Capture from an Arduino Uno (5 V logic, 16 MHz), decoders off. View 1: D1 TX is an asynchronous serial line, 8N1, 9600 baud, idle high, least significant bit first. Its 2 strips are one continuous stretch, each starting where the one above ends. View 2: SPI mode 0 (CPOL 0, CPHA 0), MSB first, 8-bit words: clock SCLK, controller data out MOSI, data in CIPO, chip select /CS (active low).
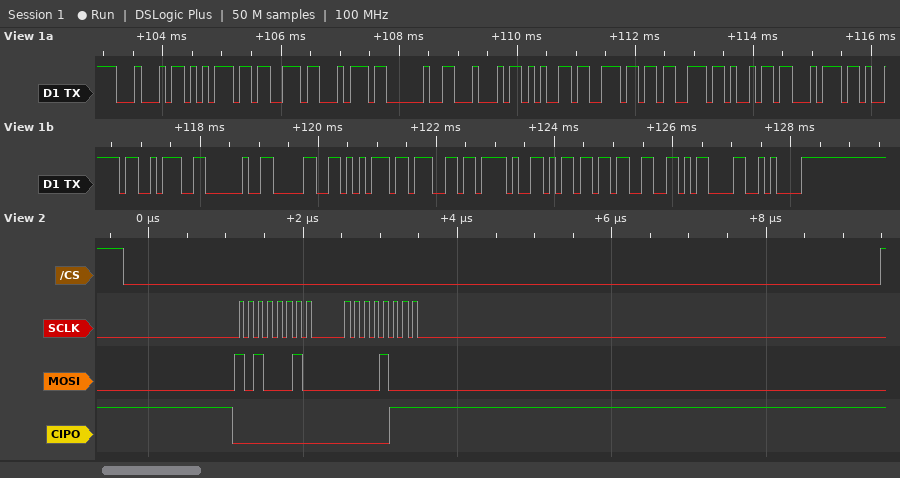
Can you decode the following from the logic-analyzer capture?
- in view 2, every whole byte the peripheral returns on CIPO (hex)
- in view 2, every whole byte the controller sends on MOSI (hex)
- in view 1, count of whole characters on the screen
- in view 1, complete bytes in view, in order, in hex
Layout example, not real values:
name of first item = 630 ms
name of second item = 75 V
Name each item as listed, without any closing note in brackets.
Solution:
in view 2, every whole byte the peripheral returns on CIPO = 00 07
in view 2, every whole byte the controller sends on MOSI = A2 08
in view 1, count of whole characters on the screen = 22
in view 1, complete bytes in view, in order, in hex = 44 75 73 74 20 44 65 6E 73 69 74 79 3A 20 30 75 67 2F 6D 33 0D 0A
